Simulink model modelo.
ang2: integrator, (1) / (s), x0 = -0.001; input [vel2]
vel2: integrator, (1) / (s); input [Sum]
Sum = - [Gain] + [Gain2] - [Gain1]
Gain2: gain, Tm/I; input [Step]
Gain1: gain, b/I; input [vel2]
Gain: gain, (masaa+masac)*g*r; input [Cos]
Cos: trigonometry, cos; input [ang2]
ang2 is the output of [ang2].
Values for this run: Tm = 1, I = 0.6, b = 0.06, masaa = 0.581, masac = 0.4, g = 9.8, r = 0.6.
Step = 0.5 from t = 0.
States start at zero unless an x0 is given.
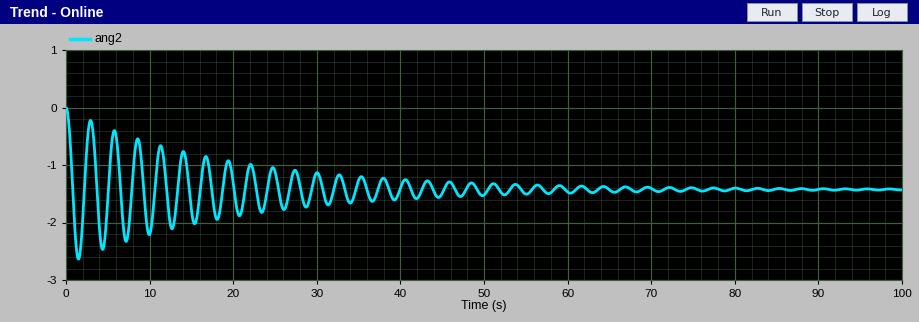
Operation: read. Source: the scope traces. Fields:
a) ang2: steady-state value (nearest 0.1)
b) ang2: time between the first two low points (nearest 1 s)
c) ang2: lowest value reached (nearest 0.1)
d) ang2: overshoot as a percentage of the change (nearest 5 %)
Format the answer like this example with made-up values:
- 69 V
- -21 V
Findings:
- -1.4
- 3 s
- -2.6
- 85 %
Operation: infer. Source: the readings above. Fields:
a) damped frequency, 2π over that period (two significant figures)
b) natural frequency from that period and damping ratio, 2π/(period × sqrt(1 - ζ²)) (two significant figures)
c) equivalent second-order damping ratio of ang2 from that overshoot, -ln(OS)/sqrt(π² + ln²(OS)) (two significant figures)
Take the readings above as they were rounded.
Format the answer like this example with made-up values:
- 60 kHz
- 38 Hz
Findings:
- 2.1 rad/s
- 2.1 rad/s
- 0.052
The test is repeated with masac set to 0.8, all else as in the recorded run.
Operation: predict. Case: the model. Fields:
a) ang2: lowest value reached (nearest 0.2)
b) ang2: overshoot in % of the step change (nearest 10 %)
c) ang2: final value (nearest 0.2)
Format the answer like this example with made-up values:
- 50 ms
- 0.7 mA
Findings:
- -2.8
- 90 %
- -1.4
